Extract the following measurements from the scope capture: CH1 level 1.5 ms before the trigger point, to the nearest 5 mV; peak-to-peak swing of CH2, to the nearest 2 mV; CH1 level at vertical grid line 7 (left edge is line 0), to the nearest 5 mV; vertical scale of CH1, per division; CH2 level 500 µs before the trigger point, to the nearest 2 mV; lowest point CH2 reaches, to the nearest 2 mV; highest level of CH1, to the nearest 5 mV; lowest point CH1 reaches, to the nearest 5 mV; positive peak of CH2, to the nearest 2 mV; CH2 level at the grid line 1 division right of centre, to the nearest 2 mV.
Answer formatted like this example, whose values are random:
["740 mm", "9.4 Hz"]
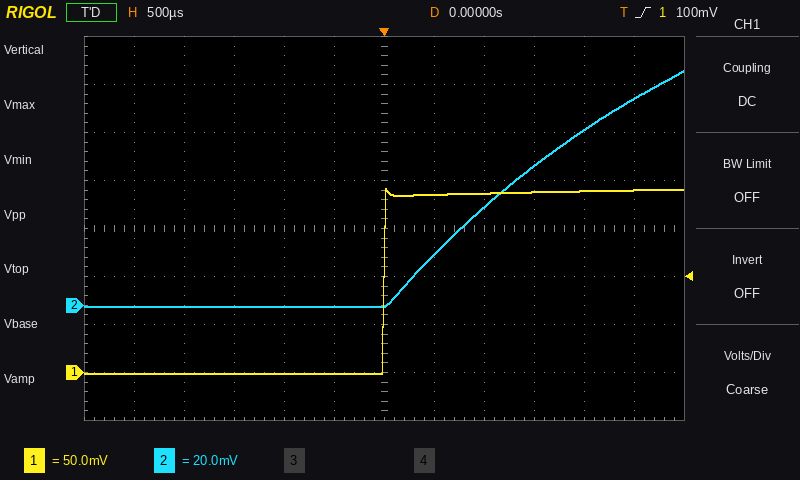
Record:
["0 mV", "98 mV", "185 mV", "50 mV", "0 mV", "0 mV", "190 mV", "0 mV", "98 mV", "22 mV"]
